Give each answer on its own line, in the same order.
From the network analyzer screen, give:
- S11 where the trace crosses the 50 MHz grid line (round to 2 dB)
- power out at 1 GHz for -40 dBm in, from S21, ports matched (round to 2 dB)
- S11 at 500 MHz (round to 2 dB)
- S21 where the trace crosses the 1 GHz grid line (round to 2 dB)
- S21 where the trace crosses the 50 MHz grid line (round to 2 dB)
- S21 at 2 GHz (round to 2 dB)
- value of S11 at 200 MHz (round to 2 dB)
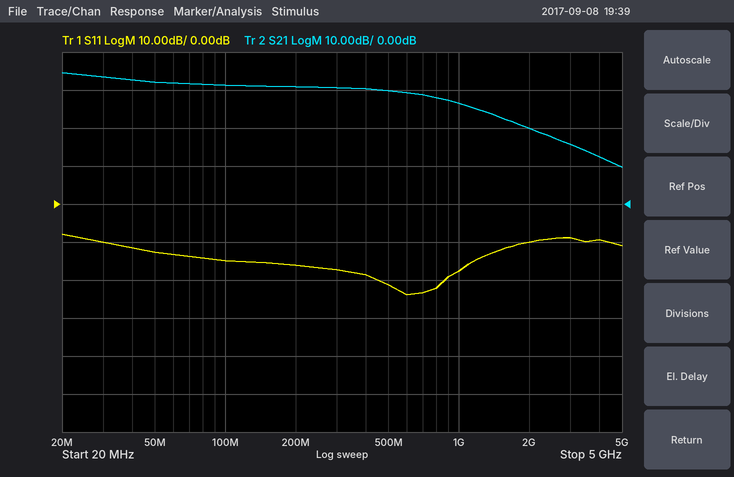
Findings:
-12 dB
-14 dBm
-22 dB
26 dB
32 dB
20 dB
-16 dB
